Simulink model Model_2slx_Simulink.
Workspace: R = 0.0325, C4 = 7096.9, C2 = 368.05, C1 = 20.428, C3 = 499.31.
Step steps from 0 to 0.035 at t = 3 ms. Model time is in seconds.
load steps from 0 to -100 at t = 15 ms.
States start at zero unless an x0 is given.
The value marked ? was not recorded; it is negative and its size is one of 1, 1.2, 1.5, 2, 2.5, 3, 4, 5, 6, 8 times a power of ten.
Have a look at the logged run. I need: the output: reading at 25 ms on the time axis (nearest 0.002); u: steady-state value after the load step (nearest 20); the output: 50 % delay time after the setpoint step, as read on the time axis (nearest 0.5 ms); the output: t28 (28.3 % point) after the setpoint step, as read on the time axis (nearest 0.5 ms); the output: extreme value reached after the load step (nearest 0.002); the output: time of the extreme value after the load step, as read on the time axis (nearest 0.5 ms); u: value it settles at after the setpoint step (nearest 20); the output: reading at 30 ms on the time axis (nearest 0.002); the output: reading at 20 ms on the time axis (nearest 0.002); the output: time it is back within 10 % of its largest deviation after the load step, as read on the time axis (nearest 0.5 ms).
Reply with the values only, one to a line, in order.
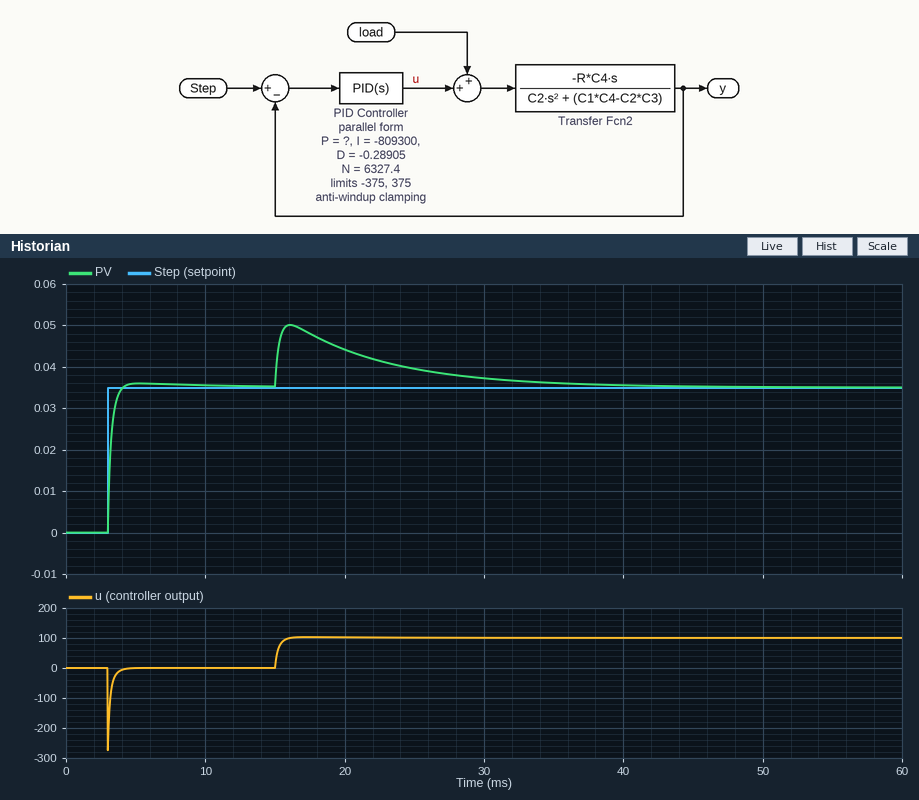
0.040
100
3.0 ms
3.0 ms
0.050
16.0 ms
0
0.038
0.044
33.0 ms
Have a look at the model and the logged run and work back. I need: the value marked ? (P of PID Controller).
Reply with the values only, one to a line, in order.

-6000
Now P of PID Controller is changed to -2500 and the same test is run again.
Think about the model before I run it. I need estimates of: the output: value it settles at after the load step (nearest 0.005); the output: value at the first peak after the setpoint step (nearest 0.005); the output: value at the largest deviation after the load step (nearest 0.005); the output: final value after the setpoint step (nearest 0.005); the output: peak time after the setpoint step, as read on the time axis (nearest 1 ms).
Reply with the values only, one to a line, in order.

0.035
0.040
0.065
0.035
6 ms
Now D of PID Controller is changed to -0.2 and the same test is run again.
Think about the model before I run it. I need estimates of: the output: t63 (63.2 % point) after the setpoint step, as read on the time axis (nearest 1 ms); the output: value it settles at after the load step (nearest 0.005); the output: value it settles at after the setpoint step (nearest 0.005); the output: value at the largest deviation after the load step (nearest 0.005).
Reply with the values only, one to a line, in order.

3 ms
0.035
0.035
0.050
